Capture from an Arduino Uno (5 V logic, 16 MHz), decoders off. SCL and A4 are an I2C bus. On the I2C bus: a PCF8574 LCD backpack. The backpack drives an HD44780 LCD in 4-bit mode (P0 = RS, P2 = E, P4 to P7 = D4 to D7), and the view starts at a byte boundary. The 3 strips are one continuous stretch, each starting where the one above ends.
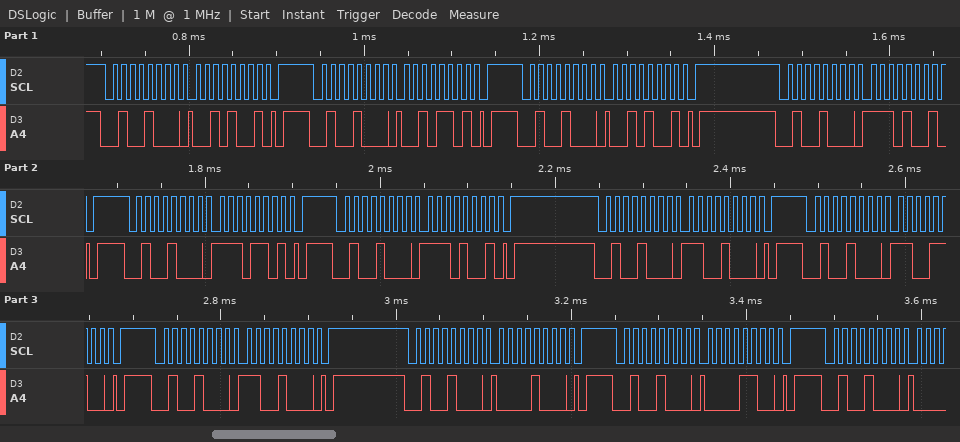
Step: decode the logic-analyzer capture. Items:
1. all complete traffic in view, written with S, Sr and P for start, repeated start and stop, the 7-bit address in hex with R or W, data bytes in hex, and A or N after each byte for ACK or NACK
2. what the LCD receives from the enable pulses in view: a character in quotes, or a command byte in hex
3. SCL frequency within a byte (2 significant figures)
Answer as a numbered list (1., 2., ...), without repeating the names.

1. S 24W A 29 A P S 24W A 2D A P S 24W A 29 A P S 24W A E9 A P S 24W A ED A P S 24W A E9 A P S 24W A C8 A P S 24W A CC A P S 24W A C8 A P S 24W A 08 A P S 24W A 0C A P S 24W A
2. '.'
3. 100 kHz
